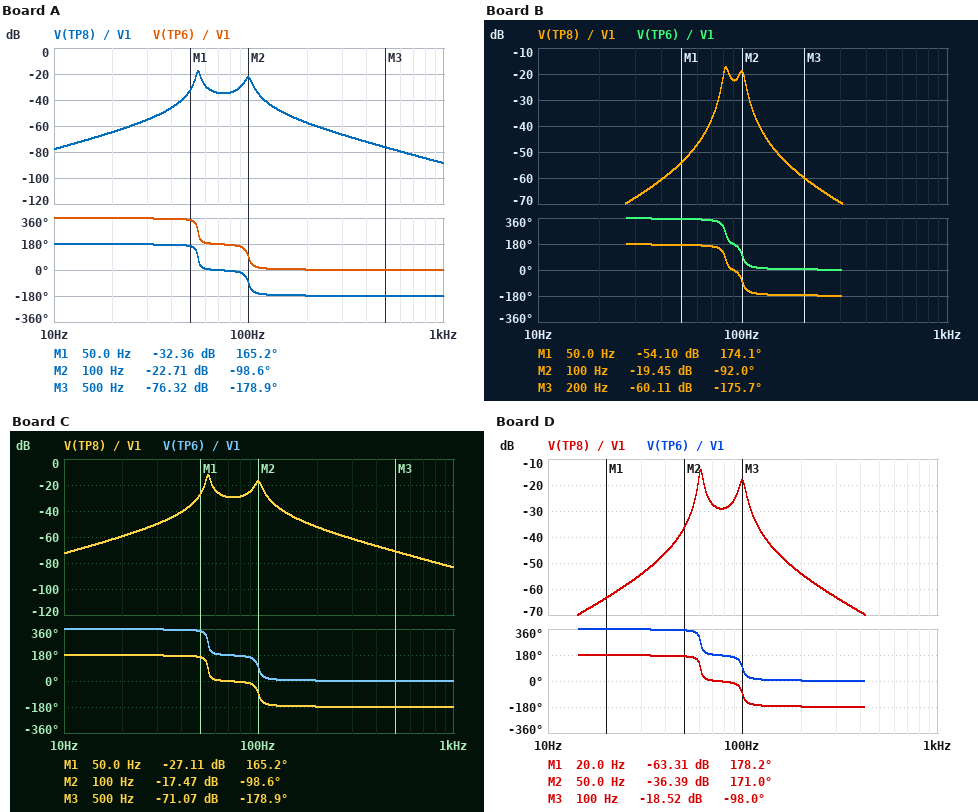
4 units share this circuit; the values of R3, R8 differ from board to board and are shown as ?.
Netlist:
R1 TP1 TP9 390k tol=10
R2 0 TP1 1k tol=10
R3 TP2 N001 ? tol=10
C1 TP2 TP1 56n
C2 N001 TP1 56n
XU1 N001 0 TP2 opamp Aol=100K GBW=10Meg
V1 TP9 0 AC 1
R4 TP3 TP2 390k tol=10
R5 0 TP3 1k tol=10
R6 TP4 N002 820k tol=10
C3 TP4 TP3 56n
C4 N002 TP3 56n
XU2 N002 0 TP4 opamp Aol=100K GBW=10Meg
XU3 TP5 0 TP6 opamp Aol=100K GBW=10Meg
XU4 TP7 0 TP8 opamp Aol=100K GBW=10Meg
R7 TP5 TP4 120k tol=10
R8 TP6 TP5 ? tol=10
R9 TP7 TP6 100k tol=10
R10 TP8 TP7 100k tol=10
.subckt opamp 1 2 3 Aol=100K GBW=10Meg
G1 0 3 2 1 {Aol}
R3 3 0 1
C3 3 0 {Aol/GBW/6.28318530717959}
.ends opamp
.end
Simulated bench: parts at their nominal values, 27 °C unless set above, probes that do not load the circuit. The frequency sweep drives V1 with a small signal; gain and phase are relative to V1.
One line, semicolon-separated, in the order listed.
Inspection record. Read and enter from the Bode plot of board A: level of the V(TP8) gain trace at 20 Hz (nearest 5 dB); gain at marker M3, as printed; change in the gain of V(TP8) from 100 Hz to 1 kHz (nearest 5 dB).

-65 dB; -76.32 dB; -65 dB
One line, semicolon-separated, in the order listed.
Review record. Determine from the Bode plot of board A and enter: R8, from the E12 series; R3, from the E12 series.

82 kΩ; 2.7 MΩ
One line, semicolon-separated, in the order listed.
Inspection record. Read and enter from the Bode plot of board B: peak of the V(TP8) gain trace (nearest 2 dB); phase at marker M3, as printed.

-18 dB; -175.7 deg
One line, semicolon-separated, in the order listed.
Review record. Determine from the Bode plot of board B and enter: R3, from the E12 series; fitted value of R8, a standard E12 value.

1.2 MΩ; 56 kΩ
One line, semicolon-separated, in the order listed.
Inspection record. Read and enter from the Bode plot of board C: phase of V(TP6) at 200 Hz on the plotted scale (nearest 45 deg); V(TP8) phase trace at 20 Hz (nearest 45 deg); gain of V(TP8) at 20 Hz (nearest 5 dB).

0 deg; 180 deg; -60 dB
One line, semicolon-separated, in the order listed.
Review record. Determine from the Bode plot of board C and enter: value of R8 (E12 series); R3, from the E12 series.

150 kΩ; 2.7 MΩ
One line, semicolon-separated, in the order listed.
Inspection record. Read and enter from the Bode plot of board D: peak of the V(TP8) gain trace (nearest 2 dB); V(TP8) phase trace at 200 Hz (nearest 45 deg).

-14 dB; -180 deg
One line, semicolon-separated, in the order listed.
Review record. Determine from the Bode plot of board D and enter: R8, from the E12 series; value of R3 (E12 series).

120 kΩ; 2.2 MΩ
